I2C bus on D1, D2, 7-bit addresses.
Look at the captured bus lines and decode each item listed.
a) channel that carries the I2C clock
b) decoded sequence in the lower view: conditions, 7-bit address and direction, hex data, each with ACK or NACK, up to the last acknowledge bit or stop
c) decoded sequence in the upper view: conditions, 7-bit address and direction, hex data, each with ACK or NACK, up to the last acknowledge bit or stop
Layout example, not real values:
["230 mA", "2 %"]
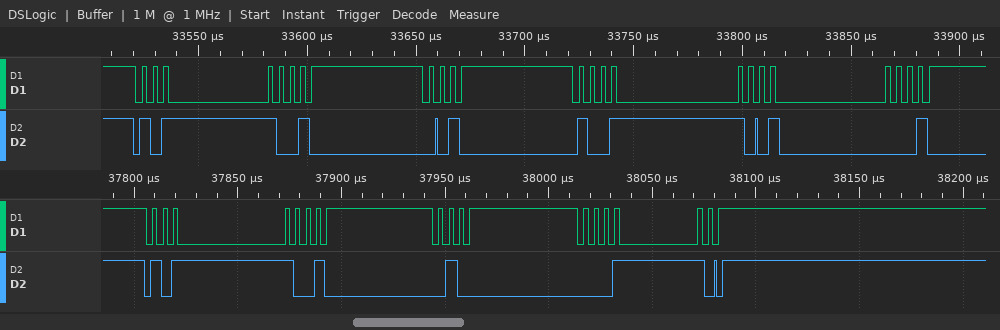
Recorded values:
["D1", "start, address 59 write ACK, 83 ACK, stop", "start, address 59 write ACK, 53 ACK"]
